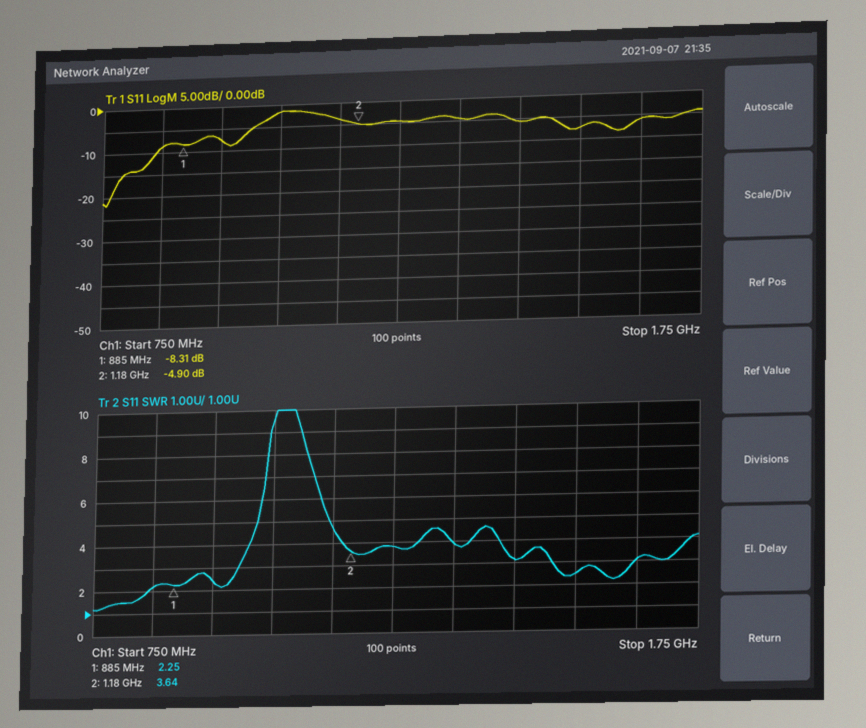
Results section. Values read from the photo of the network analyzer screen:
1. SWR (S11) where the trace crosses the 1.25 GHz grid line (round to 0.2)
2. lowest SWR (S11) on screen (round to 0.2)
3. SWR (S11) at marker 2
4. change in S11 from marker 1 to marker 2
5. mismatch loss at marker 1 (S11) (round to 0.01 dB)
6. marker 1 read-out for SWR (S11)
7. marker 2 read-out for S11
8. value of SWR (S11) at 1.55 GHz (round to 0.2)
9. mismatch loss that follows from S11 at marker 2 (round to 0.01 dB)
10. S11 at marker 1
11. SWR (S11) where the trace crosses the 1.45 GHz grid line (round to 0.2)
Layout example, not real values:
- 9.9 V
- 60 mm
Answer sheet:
- 3.8
- 1.2
- 3.64
- 3.41 dB
- 0.69 dB
- 2.25
- -4.90 dB
- 2.4
- 1.70 dB
- -8.31 dB
- 3.2
